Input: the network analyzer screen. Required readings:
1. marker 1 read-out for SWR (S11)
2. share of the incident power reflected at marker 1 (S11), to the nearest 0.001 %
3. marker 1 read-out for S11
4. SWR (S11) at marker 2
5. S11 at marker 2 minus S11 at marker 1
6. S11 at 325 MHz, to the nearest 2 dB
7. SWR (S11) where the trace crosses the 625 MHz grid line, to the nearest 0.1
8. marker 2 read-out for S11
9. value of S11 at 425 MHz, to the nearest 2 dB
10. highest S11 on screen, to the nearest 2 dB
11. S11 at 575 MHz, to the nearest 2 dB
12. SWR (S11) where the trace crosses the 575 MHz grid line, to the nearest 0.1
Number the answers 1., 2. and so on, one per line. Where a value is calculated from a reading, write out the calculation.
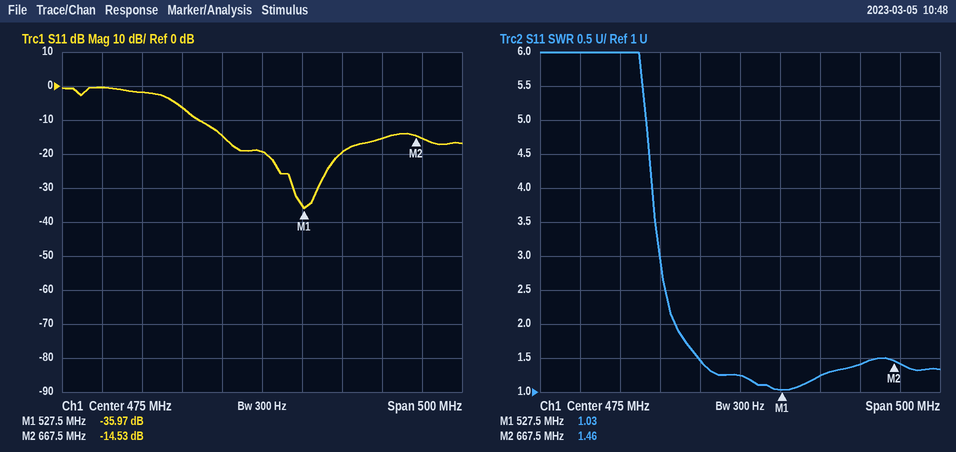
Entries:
1. 1.03
2. 10^(-35.97/10) ≈ 0.025 %
3. -35.97 dB
4. 1.46
5. -14.53 − (-35.97) = 21.44 dB
6. -2 dB
7. 1.4
8. -14.53 dB
9. -14 dB
10. 0 dB
11. -20 dB
12. 1.2
